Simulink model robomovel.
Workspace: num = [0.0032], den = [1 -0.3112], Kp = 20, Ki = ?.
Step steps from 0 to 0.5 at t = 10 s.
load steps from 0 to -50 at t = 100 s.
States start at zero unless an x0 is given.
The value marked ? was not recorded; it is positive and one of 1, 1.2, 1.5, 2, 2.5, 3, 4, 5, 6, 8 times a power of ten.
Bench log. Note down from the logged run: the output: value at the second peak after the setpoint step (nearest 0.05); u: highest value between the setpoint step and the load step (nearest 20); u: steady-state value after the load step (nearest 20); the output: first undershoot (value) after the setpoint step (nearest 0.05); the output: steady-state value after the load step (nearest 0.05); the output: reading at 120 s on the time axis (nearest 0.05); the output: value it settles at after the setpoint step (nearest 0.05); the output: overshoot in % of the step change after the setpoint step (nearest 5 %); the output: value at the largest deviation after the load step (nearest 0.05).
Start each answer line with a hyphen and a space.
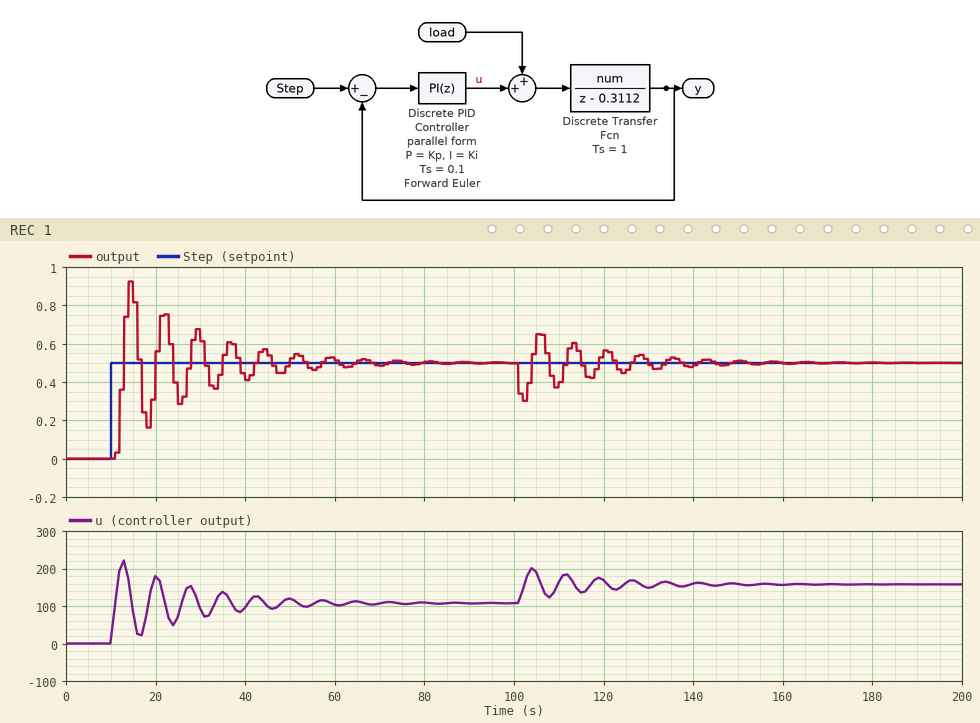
- 0.75
- 220
- 160
- 0.15
- 0.50
- 0.55
- 0.50
- 85 %
- 0.30
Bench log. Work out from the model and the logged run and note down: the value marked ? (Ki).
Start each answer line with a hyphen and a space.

- 200
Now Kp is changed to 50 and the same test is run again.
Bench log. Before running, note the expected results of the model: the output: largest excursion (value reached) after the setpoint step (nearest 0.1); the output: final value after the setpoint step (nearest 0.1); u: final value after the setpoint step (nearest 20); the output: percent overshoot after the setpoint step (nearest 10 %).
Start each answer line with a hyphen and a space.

- 0.8
- 0.5
- 100
- 70 %
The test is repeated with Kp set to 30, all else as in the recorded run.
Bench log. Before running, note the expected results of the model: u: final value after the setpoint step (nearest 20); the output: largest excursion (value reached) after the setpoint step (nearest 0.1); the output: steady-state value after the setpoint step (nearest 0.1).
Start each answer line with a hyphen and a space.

- 100
- 0.9
- 0.5
